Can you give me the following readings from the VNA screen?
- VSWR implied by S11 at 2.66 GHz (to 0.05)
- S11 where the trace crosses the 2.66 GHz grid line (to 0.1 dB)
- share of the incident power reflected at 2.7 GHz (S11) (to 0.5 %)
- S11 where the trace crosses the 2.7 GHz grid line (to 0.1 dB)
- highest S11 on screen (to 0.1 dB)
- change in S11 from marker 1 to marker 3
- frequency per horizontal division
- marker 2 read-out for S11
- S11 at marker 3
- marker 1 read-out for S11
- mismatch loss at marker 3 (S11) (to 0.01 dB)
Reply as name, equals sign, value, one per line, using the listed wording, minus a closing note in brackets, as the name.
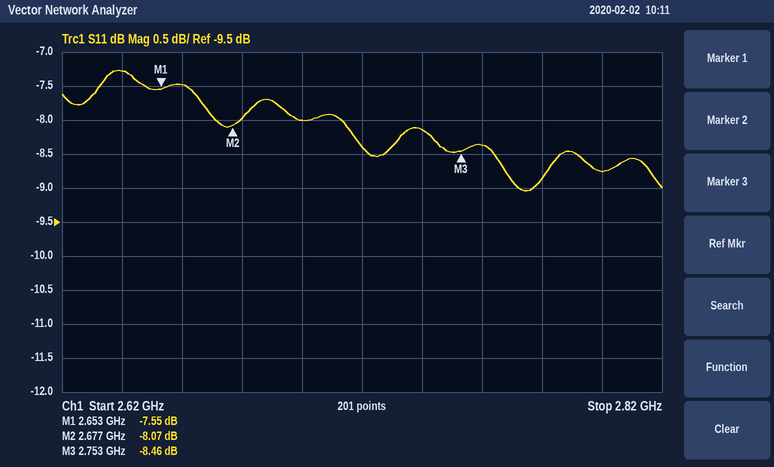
VSWR implied by S11 at 2.66 GHz = 2.45
S11 where the trace crosses the 2.66 GHz grid line = -7.5 dB
share of the incident power reflected at 2.7 GHz (S11) = 16.0 %
S11 where the trace crosses the 2.7 GHz grid line = -8.0 dB
highest S11 on screen = -7.3 dB
change in S11 from marker 1 to marker 3 = -0.91 dB
frequency per horizontal division = 20 MHz
marker 2 read-out for S11 = -8.07 dB
S11 at marker 3 = -8.46 dB
marker 1 read-out for S11 = -7.55 dB
mismatch loss at marker 3 (S11) = 0.67 dB
